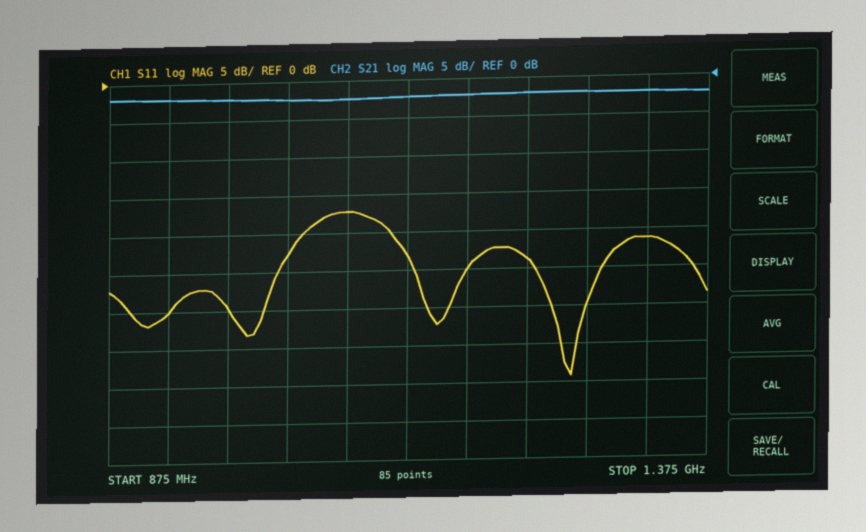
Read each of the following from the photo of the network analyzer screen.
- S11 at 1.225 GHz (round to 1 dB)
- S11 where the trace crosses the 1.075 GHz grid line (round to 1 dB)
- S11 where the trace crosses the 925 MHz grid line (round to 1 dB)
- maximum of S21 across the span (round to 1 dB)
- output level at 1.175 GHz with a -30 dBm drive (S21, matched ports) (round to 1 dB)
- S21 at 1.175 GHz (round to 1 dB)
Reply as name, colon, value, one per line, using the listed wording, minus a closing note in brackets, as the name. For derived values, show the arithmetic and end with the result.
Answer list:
S11 at 1.225 GHz: -24 dB
S11 where the trace crosses the 1.075 GHz grid line: -17 dB
S11 where the trace crosses the 925 MHz grid line: -30 dB
maximum of S21 across the span: -2 dB
output level at 1.175 GHz with a -30 dBm drive (S21, matched ports): -30 dBm + (-2 dB) = -32 dBm
S21 at 1.175 GHz: -2 dB
